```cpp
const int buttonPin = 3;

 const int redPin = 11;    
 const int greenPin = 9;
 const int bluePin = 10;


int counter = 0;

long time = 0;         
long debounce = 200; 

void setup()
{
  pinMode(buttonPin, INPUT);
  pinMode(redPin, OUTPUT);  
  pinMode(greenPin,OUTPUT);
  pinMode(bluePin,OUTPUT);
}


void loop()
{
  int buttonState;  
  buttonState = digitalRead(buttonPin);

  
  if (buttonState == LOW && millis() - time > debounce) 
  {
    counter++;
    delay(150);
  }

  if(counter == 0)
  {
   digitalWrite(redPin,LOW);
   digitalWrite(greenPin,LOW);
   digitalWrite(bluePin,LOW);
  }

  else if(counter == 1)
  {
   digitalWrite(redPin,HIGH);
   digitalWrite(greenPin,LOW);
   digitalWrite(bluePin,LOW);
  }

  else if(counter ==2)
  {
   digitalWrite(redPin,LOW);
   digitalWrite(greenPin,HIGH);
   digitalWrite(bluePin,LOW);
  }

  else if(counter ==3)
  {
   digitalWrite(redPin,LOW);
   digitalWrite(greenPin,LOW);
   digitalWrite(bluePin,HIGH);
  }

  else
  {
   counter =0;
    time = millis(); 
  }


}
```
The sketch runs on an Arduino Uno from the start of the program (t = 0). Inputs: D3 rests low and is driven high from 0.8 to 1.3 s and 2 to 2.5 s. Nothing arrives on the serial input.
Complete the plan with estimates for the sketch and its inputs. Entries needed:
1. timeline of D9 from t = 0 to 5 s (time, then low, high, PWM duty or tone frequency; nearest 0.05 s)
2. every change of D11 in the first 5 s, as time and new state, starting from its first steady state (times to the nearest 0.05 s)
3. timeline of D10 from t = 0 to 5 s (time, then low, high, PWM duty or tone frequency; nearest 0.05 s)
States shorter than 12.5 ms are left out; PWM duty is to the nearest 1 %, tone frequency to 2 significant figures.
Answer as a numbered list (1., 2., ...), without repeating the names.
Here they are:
1. 0 s low; 0.5 s high; 0.65 s low; 1.6 s high; 1.75 s low; 2.8 s high; 2.95 s low; 3.6 s high; 3.75 s low; 4.4 s high; 4.55 s low
2. 0 s low; 0.35 s high; 0.5 s low; 1.45 s high; 1.6 s low; 2.65 s high; 2.8 s low; 3.45 s high; 3.6 s low; 4.25 s high; 4.4 s low
3. 0 s low; 0.65 s high; 0.8 s low; 1.75 s high; 1.9 s low; 2.95 s high; 3.1 s low; 3.75 s high; 3.9 s low; 4.55 s high; 4.7 s low
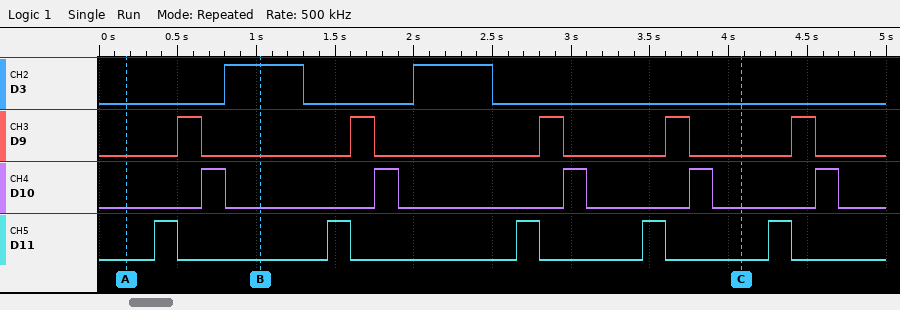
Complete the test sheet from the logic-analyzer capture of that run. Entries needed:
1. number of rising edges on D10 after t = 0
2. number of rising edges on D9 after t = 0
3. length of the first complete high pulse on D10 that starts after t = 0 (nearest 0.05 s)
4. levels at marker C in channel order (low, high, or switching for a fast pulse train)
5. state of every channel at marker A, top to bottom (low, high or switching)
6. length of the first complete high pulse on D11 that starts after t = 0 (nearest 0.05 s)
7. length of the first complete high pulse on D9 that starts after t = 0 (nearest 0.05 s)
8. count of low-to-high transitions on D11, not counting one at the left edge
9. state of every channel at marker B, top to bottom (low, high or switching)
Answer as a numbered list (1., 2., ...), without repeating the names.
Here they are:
1. 5
2. 5
3. 0.15 s
4. D3 low, D9 low, D10 low, D11 low
5. D3 low, D9 low, D10 low, D11 low
6. 0.15 s
7. 0.15 s
8. 5
9. D3 high, D9 low, D10 low, D11 low
